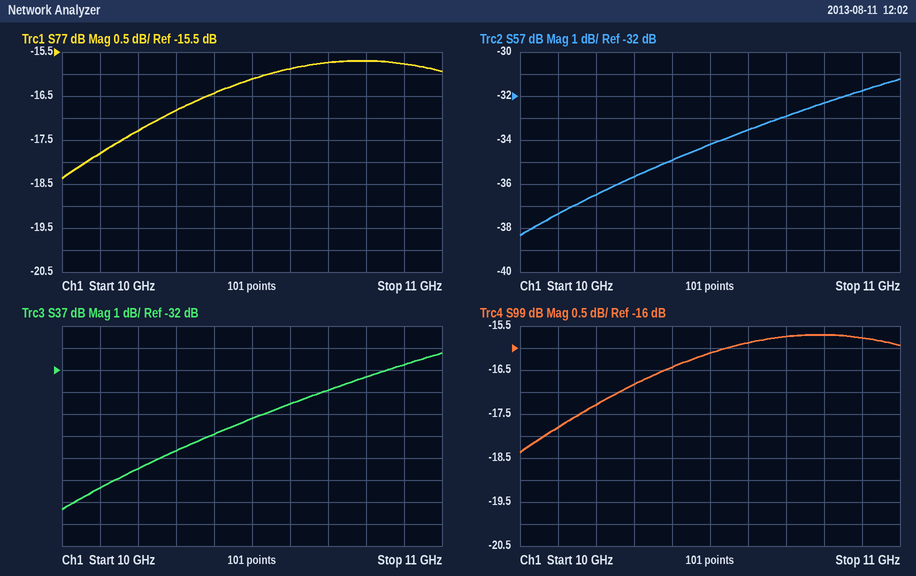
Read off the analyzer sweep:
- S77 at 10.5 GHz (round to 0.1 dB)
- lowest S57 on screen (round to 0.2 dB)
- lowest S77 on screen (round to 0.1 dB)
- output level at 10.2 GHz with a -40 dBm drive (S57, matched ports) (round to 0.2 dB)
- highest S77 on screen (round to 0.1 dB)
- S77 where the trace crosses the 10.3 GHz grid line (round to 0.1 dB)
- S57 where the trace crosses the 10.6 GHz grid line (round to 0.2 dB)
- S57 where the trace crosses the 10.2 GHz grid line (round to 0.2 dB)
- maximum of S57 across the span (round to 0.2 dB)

-16.1 dB
-38.4 dB
-18.4 dB
-76.4 dBm
-15.7 dB
-16.8 dB
-33.6 dB
-36.4 dB
-31.2 dB
